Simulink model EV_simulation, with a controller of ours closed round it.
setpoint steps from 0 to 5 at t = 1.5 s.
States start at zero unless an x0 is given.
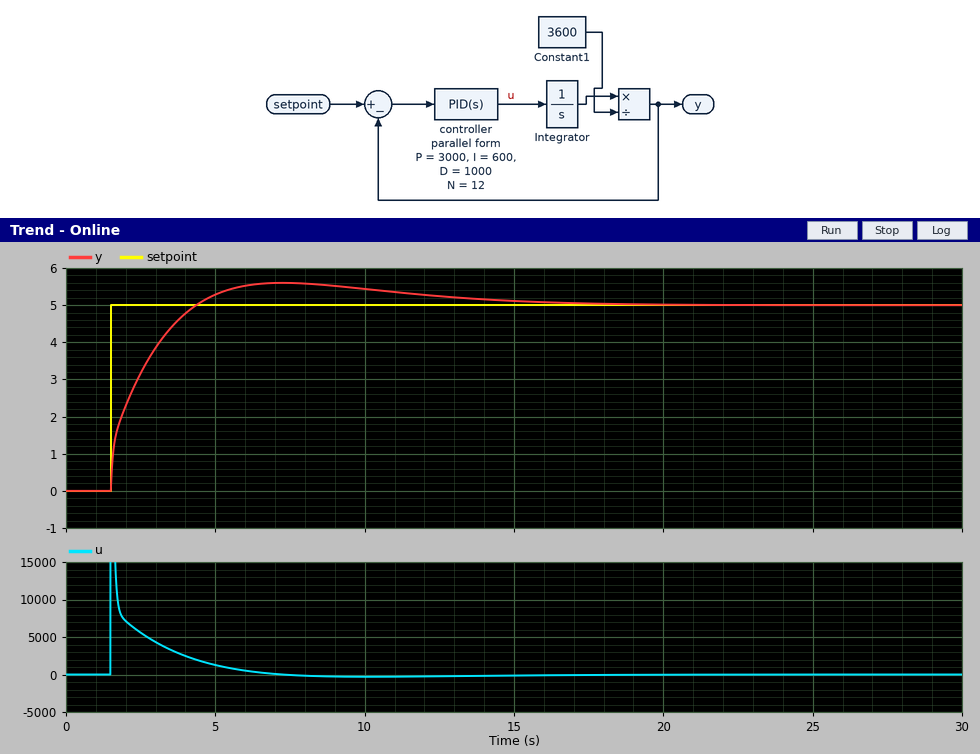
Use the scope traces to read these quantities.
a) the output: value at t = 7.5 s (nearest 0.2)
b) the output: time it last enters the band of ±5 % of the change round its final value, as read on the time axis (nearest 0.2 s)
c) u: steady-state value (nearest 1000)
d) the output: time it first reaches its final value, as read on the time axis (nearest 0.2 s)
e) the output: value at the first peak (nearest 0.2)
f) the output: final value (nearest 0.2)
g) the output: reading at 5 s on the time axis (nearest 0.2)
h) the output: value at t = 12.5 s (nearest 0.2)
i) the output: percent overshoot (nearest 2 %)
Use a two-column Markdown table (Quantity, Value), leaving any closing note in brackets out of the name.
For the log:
| Quantity | Value |
|---|---|
| the output: value at t = 7.5 s | 5.6 |
| the output: time it last enters the band of ±5 % of the change round its final value, as read on the time axis | 12.4 s |
| u: steady-state value | 0 |
| the output: time it first reaches its final value, as read on the time axis | 4.4 s |
| the output: value at the first peak | 5.6 |
| the output: final value | 5.0 |
| the output: reading at 5 s on the time axis | 5.2 |
| the output: value at t = 12.5 s | 5.2 |
| the output: percent overshoot | 12 % |
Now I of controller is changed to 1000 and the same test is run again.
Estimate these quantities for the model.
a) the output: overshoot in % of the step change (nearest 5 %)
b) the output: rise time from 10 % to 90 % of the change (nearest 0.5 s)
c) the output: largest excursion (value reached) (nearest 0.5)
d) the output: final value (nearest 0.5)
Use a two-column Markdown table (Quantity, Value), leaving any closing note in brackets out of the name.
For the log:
| Quantity | Value |
|---|---|
| the output: overshoot in % of the step change | 15 % |
| the output: rise time from 10 % to 90 % of the change | 2.0 s |
| the output: largest excursion (value reached) | 6.0 |
| the output: final value | 5.0 |
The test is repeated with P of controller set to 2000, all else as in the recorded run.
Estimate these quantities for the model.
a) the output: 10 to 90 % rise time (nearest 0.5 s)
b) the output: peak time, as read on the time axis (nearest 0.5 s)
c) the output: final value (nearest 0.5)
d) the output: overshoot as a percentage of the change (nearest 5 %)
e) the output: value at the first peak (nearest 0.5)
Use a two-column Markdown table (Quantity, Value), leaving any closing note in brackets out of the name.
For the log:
| Quantity | Value |
|---|---|
| the output: 10 to 90 % rise time | 2.5 s |
| the output: peak time, as read on the time axis | 8.0 s |
| the output: final value | 5.0 |
| the output: overshoot as a percentage of the change | 20 % |
| the output: value at the first peak | 6.0 |
